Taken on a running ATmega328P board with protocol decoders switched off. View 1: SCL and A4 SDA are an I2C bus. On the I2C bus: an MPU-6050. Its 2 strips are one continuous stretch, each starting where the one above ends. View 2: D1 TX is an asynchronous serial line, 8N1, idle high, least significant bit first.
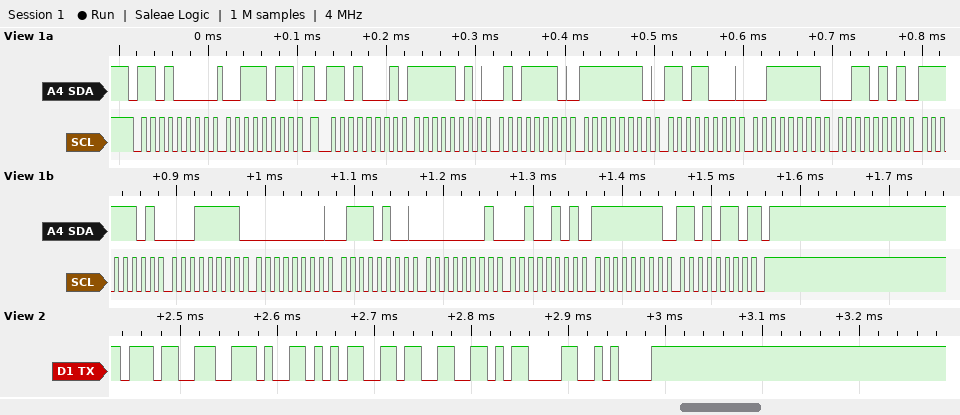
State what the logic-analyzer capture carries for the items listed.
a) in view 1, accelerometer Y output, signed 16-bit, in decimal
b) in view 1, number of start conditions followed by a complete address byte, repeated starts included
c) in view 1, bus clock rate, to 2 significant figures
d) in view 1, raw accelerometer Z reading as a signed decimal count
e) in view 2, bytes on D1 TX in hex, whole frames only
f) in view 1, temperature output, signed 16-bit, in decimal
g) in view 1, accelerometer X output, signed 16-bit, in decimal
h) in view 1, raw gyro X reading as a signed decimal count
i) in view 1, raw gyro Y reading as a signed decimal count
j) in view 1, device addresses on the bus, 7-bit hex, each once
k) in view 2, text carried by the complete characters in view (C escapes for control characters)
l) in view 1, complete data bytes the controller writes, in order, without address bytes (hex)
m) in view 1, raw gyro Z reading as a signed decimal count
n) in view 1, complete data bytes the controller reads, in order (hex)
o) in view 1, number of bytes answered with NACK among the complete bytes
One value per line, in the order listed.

-296
2
100 kHz
16181
37 2E 35 33 0D 0A
-737
-1442
116
293
0x68
"7.53\r\n"
3B
-42
FA 5E FE D8 3F 35 FD 1F 00 74 01 25 FF D6
1
